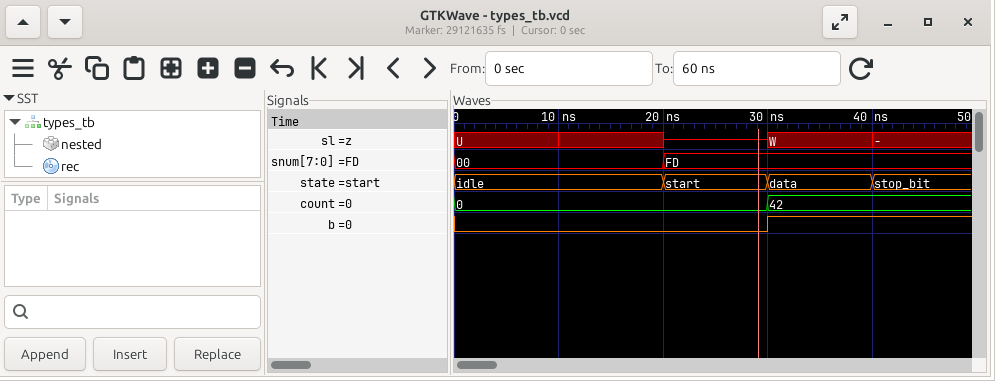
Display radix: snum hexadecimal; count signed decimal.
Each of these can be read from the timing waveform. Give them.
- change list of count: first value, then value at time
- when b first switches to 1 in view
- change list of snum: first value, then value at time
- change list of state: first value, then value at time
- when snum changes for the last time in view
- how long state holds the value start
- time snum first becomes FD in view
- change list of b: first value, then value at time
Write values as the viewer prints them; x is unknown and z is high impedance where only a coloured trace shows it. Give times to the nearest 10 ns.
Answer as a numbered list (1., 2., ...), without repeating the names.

1. 0, 42 at 30 ns
2. 30 ns
3. 00, FD at 20 ns
4. idle, start at 20 ns, data at 30 ns, stop_bit at 40 ns
5. 20 ns
6. 10 ns
7. 20 ns
8. 0, 1 at 30 ns
